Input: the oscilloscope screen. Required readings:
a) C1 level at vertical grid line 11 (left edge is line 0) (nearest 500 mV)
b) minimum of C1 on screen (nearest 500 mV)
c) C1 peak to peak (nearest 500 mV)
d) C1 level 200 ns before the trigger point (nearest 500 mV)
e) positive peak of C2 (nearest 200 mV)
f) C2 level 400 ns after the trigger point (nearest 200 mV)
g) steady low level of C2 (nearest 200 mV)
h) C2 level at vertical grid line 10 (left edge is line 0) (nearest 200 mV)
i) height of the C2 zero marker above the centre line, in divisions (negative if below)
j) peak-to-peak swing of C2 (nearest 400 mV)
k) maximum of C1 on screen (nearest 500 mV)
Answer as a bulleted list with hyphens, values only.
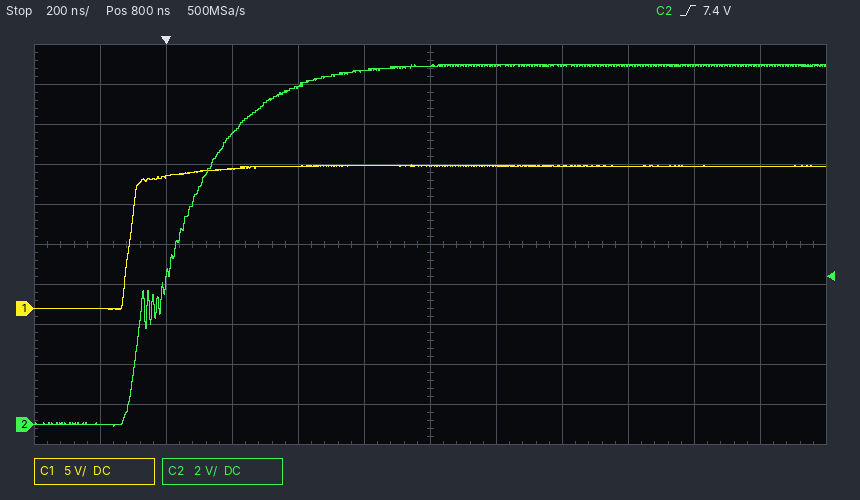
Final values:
- 18.0 V
- 0.0 V
- 18.0 V
- 0.0 V
- 18.0 V
- 17.0 V
- 0.0 V
- 18.0 V
- -4.5 div
- 18.0 V
- 18.0 V
